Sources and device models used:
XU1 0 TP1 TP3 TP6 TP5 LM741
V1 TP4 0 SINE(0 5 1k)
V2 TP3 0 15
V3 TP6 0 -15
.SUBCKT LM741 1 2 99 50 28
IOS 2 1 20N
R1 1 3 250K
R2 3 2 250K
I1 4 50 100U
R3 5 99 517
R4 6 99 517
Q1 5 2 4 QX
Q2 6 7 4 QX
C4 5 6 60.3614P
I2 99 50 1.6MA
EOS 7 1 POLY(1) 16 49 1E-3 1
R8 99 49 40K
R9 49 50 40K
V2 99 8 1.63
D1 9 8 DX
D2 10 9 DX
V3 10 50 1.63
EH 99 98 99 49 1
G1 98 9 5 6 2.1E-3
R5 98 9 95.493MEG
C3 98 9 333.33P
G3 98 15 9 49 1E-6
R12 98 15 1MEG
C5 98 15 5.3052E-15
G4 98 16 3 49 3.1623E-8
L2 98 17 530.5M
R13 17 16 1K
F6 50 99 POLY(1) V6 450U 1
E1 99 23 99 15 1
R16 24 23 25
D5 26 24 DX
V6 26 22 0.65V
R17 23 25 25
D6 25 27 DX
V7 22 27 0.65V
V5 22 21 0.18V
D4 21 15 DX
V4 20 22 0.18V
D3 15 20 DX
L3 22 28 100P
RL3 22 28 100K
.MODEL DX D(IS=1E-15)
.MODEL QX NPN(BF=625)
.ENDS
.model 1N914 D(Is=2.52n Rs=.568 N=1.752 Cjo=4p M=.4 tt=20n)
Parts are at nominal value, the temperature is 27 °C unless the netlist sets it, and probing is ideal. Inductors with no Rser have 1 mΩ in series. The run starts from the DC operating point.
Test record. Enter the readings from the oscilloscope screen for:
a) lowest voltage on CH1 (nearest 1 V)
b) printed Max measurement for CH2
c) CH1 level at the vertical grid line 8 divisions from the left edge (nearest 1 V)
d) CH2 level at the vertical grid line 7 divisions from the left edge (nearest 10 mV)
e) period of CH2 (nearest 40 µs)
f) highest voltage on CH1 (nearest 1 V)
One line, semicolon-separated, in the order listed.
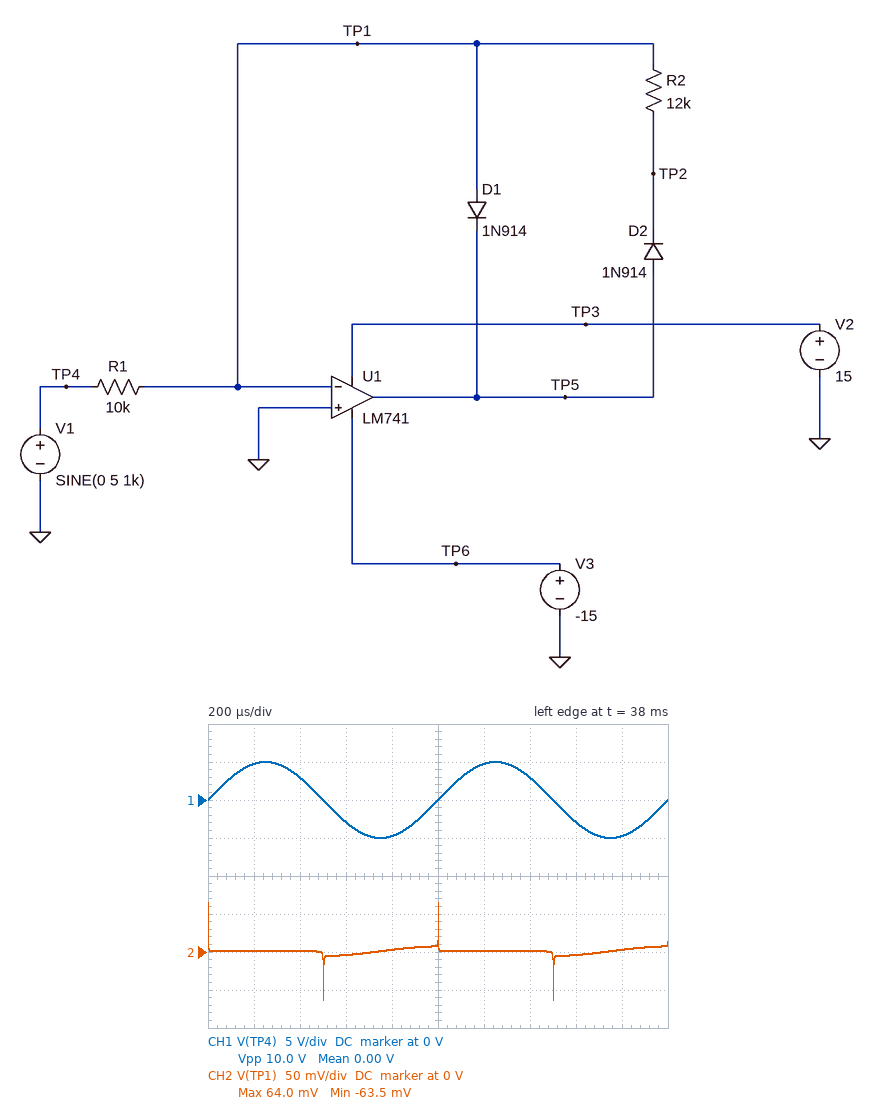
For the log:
-5 V; 64.0 mV; -3 V; 0 V; 1.00 ms; 5 V
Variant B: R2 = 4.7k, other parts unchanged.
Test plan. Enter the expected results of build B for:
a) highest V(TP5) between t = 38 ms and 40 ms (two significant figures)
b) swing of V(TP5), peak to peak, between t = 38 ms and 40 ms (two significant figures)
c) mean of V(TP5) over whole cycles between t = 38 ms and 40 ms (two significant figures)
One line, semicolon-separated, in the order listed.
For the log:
2.9 V; 3.5 V; 750 mV
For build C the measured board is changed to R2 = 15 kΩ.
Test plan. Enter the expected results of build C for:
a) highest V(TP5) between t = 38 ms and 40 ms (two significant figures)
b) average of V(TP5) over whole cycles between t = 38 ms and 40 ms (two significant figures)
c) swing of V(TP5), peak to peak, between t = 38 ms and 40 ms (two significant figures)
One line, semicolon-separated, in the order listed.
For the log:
8.1 V; 2.4 V; 8.6 V
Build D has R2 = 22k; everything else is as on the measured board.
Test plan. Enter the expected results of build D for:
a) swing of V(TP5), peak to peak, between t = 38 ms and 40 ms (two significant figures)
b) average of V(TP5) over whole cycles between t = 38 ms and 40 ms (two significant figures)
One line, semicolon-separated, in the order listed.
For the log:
12 V; 3.5 V
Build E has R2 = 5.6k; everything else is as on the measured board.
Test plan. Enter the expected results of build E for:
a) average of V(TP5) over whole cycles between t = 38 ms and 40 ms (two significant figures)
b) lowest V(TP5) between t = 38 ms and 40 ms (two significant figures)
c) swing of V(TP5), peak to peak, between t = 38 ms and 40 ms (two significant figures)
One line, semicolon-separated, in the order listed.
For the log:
890 mV; -550 mV; 3.9 V
